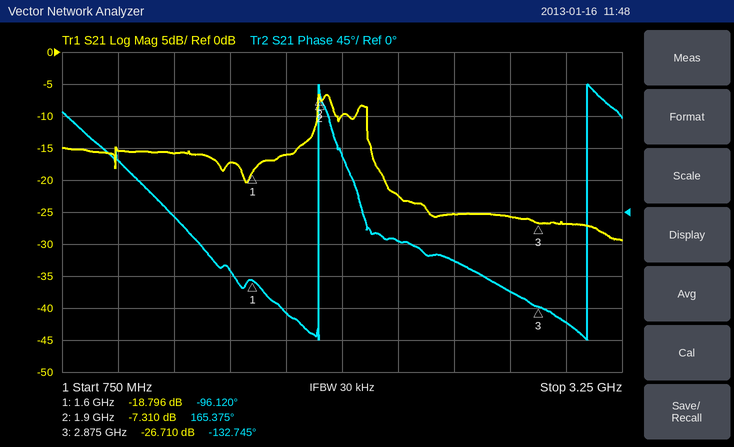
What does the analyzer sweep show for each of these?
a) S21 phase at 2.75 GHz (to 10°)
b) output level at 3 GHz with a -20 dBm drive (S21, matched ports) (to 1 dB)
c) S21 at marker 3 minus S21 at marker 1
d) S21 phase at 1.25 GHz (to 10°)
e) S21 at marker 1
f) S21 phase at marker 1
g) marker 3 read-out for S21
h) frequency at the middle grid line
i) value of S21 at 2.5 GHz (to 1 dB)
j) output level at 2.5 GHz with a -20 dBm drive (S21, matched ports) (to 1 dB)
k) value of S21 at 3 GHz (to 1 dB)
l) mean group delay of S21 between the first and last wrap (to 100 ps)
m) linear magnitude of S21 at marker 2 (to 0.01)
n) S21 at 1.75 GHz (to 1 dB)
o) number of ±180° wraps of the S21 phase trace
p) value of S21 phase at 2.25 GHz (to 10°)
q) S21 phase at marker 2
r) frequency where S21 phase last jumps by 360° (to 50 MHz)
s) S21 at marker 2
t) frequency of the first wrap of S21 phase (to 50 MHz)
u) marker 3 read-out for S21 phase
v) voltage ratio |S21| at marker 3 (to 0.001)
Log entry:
-110°
-47 dBm
-7.914 dB
-10°
-18.796 dB
-96.120°
-26.710 dB
2 GHz
-25 dB
-45 dBm
-27 dB
800 ps
0.43
-16 dB
2
-40°
165.375°
3.10 GHz
-7.310 dB
1.90 GHz
-132.745°
0.046
